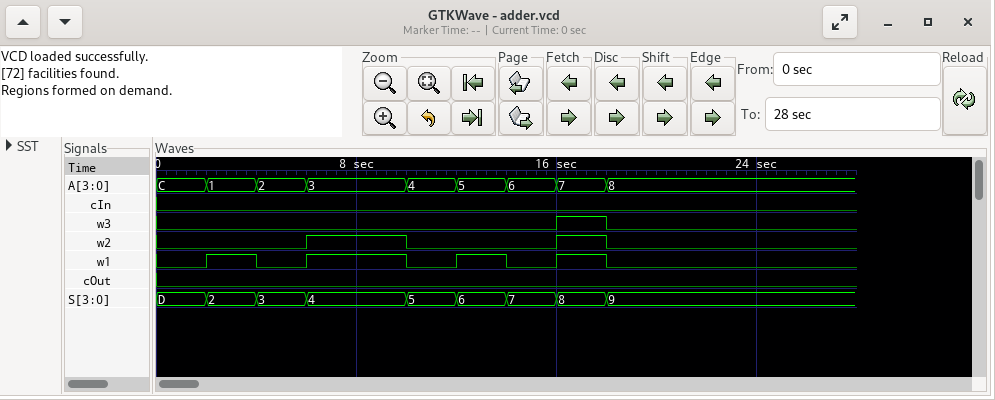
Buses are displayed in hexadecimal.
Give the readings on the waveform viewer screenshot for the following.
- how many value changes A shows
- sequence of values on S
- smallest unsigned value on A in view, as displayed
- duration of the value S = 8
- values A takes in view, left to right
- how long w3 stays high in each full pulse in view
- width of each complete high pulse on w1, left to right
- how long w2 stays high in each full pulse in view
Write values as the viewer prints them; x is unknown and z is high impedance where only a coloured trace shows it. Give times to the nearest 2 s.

8
D, 2, 3, 4, 5, 6, 7, 8, 9
1
2 s
C, 1, 2, 3, 4, 5, 6, 7, 8
2 s
2 s, 4 s, 2 s, 2 s
4 s, 2 s
